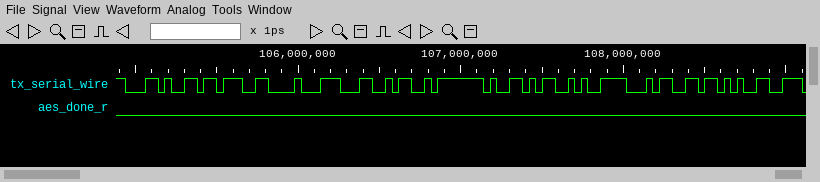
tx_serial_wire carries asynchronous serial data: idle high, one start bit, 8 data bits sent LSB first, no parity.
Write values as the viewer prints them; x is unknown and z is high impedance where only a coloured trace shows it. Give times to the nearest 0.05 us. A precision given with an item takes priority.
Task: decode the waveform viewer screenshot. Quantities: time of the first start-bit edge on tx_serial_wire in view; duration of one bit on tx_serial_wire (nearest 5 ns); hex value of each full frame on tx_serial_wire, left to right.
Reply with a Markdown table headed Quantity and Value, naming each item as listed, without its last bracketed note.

| Quantity | Value |
|---|---|
| time of the first start-bit edge on tx_serial_wire in view | 104.95 us |
| duration of one bit on tx_serial_wire | 40 ns |
| hex value of each full frame on tx_serial_wire, left to right | 2C, 3B, 88, 4C, FA, 59, CA, 34, 2B |
